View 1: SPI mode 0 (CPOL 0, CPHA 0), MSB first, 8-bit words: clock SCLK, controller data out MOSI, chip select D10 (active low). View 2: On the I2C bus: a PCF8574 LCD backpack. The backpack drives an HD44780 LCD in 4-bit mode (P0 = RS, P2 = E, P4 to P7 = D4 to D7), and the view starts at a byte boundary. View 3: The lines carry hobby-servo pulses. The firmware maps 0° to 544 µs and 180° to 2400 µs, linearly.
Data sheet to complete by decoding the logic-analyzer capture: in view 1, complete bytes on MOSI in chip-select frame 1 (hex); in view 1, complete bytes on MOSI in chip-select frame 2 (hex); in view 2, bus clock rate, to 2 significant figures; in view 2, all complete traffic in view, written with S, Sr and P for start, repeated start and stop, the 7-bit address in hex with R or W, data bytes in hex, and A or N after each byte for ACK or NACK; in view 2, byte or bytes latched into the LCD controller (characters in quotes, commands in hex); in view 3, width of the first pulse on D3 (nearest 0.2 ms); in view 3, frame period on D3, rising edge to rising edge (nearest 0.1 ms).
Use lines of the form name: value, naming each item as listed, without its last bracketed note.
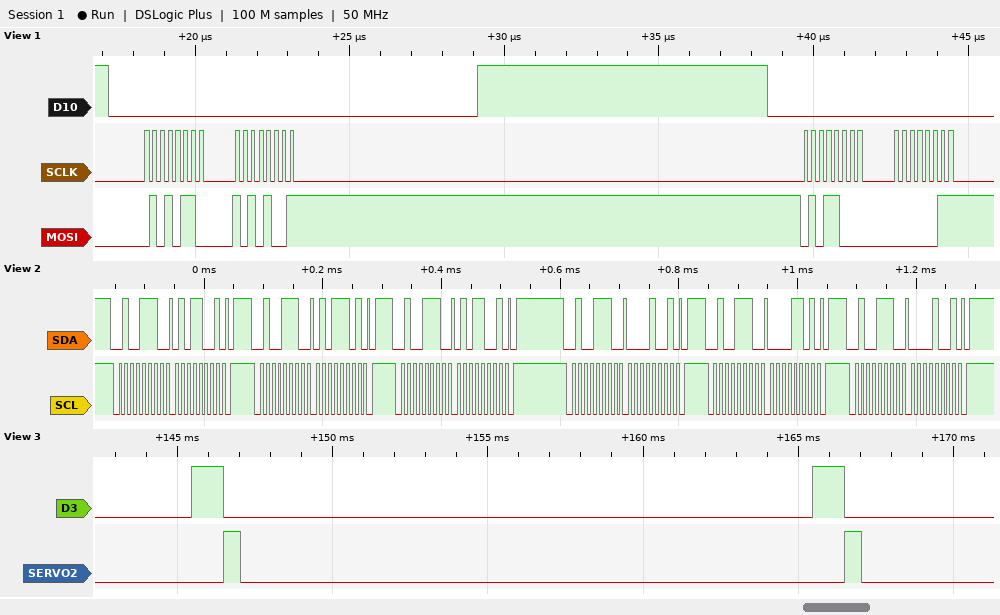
in view 1, complete bytes on MOSI in chip-select frame 1: 0x56 0xA9
in view 1, complete bytes on MOSI in chip-select frame 2: 0x58 0x03
in view 2, bus clock rate, to 2 significant figures: 100 kHz
in view 2, all complete traffic in view, written with S, Sr and P for start, repeated start and stop, the 7-bit address in hex with R or W, data bytes in hex, and A or N after each byte for ACK or NACK: S 27W A 59 A P S 27W A 5D A P S 27W A 59 A P S 27W A 09 A P S 27W A 0D A P S 27W A 09 A P
in view 2, byte or bytes latched into the LCD controller: 'P'
in view 3, width of the first pulse on D3: 1.0 ms
in view 3, frame period on D3, rising edge to rising edge: 20.0 ms
